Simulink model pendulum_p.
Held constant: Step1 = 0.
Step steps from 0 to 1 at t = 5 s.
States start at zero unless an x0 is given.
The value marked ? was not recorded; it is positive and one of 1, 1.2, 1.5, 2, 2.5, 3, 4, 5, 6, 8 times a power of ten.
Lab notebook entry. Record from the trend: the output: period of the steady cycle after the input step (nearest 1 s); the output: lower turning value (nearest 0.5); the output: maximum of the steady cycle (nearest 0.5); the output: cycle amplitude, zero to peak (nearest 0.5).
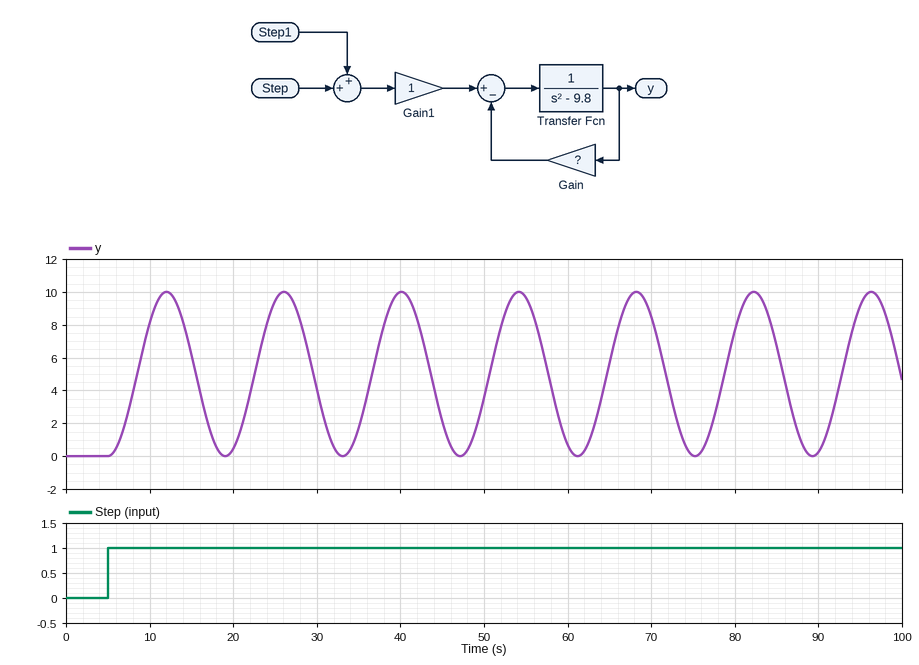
14 s
0.0
10.0
5.0
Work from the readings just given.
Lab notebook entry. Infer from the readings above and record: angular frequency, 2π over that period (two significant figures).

0.45 rad/s
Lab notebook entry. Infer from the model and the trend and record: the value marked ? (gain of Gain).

10
